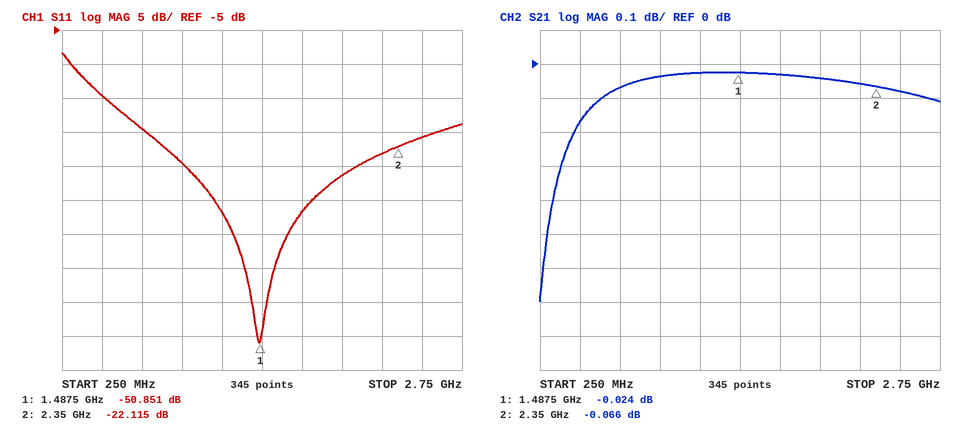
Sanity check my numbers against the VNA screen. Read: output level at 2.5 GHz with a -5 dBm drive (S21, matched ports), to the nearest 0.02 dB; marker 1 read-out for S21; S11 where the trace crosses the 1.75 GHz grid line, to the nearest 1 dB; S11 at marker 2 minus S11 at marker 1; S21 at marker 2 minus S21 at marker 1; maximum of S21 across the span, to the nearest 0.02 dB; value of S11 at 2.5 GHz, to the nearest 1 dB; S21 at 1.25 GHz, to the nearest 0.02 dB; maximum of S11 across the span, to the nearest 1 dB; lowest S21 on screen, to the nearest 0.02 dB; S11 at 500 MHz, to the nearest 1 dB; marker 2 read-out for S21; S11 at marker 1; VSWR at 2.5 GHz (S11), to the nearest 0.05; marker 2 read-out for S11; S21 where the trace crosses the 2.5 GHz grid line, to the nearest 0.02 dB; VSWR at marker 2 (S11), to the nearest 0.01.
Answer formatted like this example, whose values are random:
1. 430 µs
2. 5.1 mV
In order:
1. -5.08 dBm
2. -0.024 dB
3. -32 dB
4. 28.736 dB
5. -0.042 dB
6. -0.02 dB
7. -21 dB
8. -0.02 dB
9. -8 dB
10. -0.70 dB
11. -15 dB
12. -0.066 dB
13. -50.851 dB
14. 1.20
15. -22.115 dB
16. -0.08 dB
17. 1.17
